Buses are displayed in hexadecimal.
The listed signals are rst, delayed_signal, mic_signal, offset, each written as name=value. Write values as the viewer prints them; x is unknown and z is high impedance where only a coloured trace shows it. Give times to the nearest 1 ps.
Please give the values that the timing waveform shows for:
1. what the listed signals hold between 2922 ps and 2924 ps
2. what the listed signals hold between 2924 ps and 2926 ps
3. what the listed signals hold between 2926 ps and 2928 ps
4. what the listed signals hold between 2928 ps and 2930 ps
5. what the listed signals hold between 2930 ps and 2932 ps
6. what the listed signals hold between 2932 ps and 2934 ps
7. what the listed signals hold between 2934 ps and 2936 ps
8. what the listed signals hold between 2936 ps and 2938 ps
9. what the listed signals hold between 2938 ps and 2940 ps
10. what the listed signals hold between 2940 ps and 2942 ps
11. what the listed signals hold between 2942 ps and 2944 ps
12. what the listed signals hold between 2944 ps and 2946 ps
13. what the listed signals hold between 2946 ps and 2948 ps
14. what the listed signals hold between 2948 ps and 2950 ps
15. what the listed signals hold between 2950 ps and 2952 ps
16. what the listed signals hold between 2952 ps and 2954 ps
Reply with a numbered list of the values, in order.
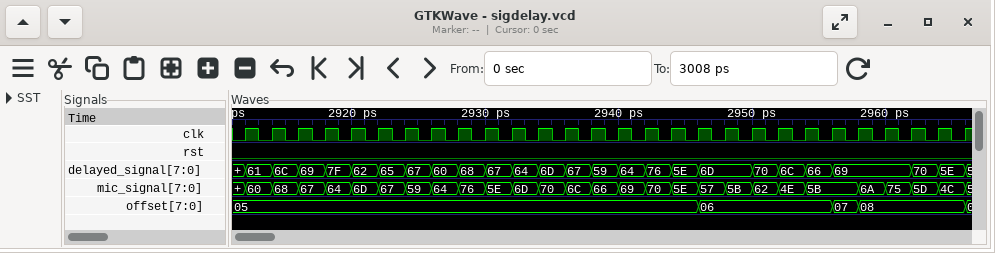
1. rst=0, delayed_signal=65, mic_signal=67, offset=05
2. rst=0, delayed_signal=67, mic_signal=59, offset=05
3. rst=0, delayed_signal=60, mic_signal=64, offset=05
4. rst=0, delayed_signal=68, mic_signal=76, offset=05
5. rst=0, delayed_signal=67, mic_signal=5E, offset=05
6. rst=0, delayed_signal=64, mic_signal=6D, offset=05
7. rst=0, delayed_signal=6D, mic_signal=70, offset=05
8. rst=0, delayed_signal=67, mic_signal=6C, offset=05
9. rst=0, delayed_signal=59, mic_signal=66, offset=05
10. rst=0, delayed_signal=64, mic_signal=69, offset=05
11. rst=0, delayed_signal=76, mic_signal=70, offset=05
12. rst=0, delayed_signal=5E, mic_signal=5E, offset=05
13. rst=0, delayed_signal=6D, mic_signal=57, offset=06
14. rst=0, delayed_signal=6D, mic_signal=5B, offset=06
15. rst=0, delayed_signal=70, mic_signal=62, offset=06
16. rst=0, delayed_signal=6C, mic_signal=4E, offset=06
